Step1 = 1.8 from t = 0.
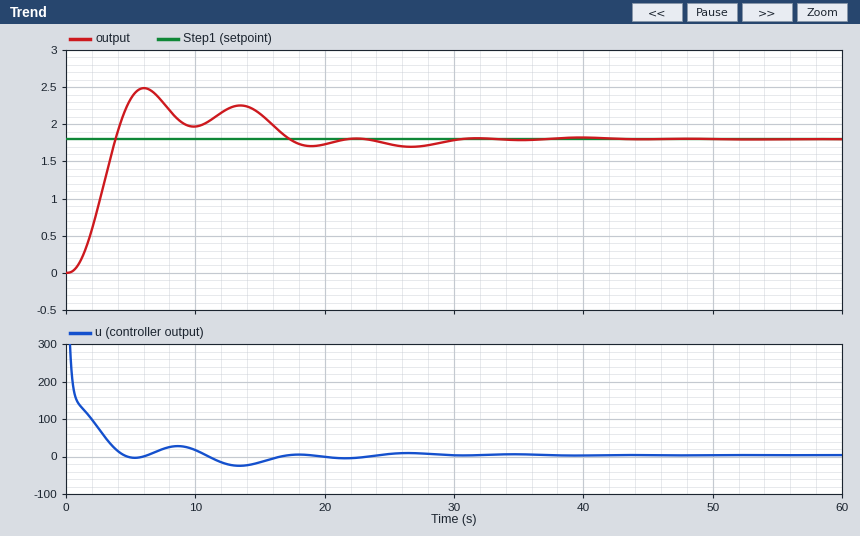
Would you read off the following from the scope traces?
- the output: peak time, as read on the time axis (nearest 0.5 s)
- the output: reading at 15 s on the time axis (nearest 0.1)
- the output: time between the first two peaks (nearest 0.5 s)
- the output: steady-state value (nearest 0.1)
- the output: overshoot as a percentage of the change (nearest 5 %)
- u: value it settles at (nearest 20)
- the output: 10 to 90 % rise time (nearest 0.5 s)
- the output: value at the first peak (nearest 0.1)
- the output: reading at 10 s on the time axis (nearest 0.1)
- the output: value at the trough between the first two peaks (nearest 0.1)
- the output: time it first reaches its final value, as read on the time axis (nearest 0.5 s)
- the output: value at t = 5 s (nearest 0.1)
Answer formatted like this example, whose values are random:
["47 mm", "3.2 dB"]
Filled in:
["6.0 s", "2.1", "7.5 s", "1.8", "40 %", "0", "2.5 s", "2.5", "2.0", "2.0", "4.0 s", "2.3"]
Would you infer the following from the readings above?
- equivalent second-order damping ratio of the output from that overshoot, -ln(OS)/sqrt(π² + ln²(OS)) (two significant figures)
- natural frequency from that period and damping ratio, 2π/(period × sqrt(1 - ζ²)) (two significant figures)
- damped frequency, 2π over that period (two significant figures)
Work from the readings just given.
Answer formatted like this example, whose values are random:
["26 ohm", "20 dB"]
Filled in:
["0.28", "0.87 rad/s", "0.84 rad/s"]
